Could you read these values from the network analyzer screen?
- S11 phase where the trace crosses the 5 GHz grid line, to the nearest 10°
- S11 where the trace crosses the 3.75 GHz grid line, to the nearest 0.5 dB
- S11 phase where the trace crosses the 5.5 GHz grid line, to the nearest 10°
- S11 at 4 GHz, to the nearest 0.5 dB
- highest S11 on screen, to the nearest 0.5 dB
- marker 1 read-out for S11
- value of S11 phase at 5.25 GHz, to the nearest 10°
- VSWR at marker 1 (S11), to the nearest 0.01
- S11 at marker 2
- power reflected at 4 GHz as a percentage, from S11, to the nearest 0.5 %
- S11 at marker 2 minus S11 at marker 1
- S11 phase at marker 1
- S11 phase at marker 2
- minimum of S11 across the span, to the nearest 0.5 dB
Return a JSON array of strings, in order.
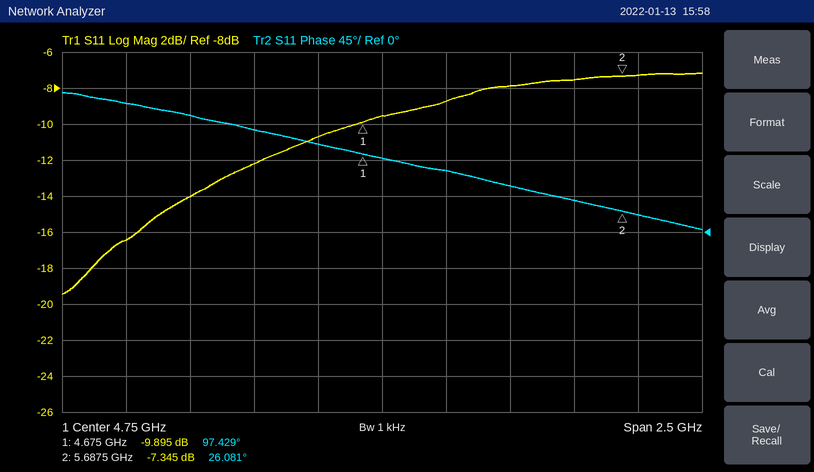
["80°", "-16.5 dB", "40°", "-14.0 dB", "-7.0 dB", "-9.895 dB", "60°", "1.94", "-7.345 dB", "4.0 %", "2.550 dB", "97.429°", "26.081°", "-19.5 dB"]
